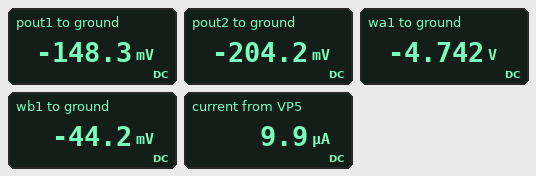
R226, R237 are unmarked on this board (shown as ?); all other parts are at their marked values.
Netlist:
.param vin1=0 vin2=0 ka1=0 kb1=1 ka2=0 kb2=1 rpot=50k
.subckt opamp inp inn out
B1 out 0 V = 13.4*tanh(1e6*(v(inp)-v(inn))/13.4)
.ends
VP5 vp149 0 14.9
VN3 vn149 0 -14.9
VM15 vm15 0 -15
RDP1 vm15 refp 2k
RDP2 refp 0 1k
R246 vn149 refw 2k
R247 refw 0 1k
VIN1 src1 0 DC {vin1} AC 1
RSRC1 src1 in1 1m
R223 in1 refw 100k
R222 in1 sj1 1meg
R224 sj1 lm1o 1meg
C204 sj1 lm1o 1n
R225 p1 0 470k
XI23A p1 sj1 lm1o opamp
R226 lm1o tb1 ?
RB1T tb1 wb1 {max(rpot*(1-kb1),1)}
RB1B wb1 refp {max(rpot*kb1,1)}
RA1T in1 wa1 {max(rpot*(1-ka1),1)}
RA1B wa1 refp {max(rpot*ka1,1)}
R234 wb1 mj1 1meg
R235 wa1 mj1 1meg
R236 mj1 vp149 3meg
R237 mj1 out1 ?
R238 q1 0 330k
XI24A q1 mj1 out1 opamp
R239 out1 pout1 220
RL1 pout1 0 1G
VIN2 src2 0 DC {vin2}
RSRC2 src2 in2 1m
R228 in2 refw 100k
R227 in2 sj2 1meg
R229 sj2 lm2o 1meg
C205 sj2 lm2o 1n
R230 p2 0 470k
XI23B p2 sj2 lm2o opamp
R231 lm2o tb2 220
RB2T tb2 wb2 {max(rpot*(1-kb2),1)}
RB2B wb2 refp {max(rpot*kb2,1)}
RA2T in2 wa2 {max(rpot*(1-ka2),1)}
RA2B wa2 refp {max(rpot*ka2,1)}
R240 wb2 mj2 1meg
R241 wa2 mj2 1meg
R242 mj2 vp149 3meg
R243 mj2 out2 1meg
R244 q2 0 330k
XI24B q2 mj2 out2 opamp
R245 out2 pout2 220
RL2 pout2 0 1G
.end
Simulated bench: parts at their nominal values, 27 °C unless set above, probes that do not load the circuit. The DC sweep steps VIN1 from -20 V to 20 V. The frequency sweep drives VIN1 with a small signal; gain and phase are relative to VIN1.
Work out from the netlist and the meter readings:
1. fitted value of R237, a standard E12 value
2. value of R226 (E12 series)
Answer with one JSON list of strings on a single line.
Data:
["820 kΩ", "470 Ω"]
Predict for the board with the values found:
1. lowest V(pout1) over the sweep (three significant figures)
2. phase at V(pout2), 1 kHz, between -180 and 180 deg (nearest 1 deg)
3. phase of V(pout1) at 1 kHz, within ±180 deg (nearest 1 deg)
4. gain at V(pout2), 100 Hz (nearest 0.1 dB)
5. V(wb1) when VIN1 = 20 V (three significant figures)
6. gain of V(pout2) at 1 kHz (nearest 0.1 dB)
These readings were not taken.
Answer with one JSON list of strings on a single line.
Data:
["-11.0 V", "-171 deg", "-86 deg", "-43.4 dB", "-13.3 V", "-38.0 dB"]
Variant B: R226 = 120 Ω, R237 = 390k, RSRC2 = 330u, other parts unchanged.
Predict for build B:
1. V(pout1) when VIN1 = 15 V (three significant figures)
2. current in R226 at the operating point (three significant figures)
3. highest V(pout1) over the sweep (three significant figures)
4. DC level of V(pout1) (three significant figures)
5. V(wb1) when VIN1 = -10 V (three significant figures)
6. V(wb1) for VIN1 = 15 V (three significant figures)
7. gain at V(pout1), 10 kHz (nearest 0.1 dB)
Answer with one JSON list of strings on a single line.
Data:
["5.12 V", "94.6 µA", "5.13 V", "-83.5 mV", "9.96 V", "-13.4 V", "-42.0 dB"]
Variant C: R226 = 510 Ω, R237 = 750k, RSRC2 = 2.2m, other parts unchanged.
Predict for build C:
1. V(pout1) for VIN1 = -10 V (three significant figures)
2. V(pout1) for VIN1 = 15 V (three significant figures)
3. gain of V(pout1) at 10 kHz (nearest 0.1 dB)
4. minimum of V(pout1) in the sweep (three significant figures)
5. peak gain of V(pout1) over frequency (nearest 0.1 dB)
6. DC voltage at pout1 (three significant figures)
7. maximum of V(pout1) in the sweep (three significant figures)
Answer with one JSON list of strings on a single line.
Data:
["-7.55 V", "9.79 V", "-36.4 dB", "-10.1 V", "-2.6 dB", "-133 mV", "9.81 V"]
